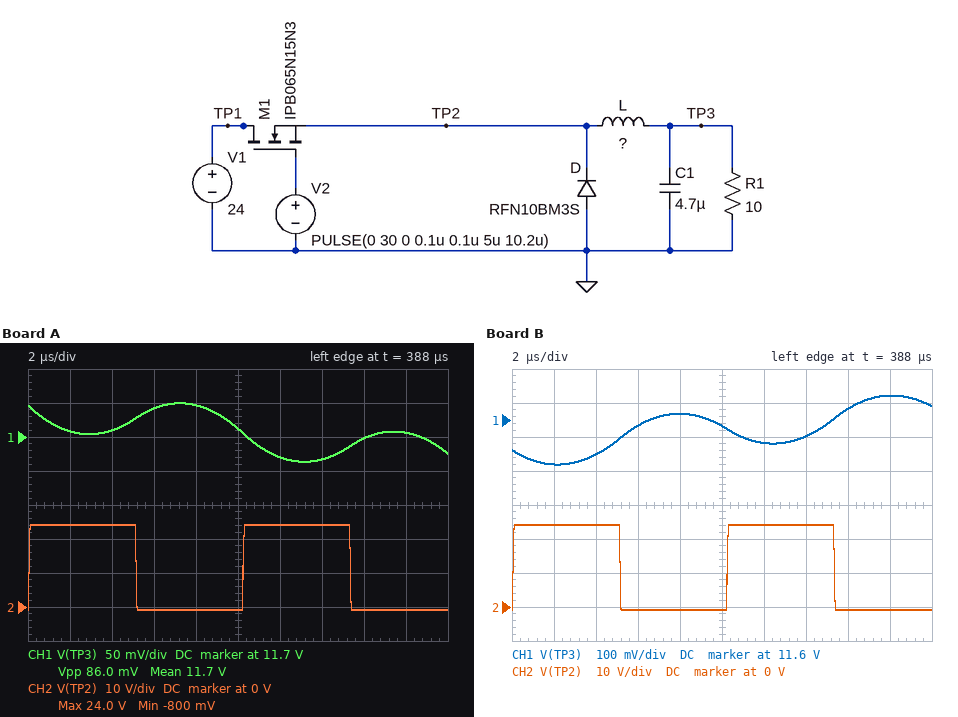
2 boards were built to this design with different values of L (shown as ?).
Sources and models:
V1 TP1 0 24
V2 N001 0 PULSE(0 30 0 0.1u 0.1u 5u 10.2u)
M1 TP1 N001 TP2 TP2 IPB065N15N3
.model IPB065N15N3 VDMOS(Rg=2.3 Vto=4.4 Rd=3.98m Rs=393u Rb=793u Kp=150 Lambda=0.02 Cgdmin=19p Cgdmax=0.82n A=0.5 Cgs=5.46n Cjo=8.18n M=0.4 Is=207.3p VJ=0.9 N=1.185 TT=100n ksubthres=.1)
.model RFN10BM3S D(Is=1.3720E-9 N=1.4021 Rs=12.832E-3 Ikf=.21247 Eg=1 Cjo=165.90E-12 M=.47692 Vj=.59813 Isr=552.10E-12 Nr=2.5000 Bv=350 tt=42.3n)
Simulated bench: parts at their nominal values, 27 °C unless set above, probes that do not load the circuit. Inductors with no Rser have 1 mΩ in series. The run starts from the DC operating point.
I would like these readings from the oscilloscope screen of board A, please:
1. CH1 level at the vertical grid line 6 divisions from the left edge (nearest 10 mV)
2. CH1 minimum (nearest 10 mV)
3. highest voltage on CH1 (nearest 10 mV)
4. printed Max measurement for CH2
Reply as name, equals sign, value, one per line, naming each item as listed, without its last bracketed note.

CH1 level at the vertical grid line 6 divisions from the left edge = 11.67 V
CH1 minimum = 11.66 V
highest voltage on CH1 = 11.75 V
printed Max measurement for CH2 = 24.0 V
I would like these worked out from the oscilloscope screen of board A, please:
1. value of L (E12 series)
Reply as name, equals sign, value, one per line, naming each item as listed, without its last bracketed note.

value of L = 270 µH
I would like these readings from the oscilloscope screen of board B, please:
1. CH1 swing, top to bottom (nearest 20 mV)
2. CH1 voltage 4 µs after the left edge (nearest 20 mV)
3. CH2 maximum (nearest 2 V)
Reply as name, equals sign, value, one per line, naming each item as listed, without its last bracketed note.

CH1 swing, top to bottom = 200 mV
CH1 voltage 4 µs after the left edge = 11.50 V
CH2 maximum = 24 V
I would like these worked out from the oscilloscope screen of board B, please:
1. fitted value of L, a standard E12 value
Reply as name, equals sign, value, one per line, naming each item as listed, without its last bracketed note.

fitted value of L, a standard E12 value = 150 µH
